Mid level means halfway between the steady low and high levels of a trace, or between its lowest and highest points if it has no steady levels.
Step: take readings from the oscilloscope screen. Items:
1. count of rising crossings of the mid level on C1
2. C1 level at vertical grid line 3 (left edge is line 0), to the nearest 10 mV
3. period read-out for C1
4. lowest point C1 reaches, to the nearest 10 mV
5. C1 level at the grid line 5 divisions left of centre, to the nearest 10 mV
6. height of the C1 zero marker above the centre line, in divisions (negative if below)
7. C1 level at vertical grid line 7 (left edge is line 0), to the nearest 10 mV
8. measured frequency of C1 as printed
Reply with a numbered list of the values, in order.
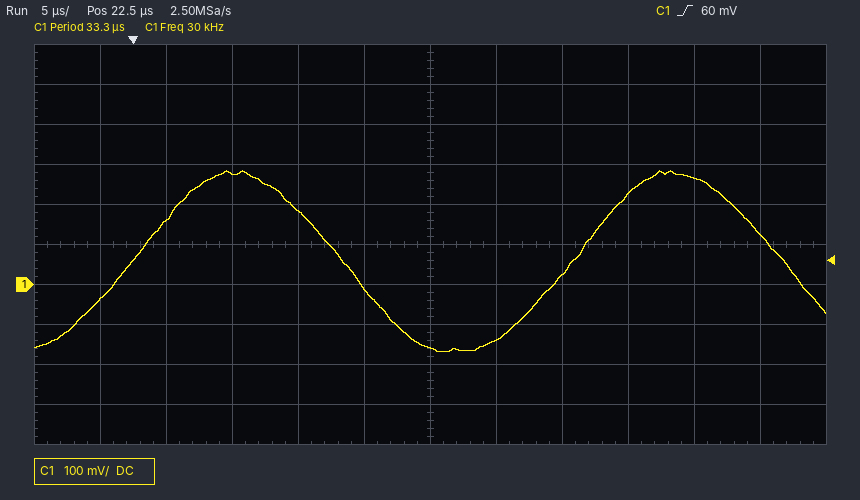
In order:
1. 2
2. 280 mV
3. 33.3 µs
4. -170 mV
5. -40 mV
6. -1.0 div
7. -140 mV
8. 30 kHz
